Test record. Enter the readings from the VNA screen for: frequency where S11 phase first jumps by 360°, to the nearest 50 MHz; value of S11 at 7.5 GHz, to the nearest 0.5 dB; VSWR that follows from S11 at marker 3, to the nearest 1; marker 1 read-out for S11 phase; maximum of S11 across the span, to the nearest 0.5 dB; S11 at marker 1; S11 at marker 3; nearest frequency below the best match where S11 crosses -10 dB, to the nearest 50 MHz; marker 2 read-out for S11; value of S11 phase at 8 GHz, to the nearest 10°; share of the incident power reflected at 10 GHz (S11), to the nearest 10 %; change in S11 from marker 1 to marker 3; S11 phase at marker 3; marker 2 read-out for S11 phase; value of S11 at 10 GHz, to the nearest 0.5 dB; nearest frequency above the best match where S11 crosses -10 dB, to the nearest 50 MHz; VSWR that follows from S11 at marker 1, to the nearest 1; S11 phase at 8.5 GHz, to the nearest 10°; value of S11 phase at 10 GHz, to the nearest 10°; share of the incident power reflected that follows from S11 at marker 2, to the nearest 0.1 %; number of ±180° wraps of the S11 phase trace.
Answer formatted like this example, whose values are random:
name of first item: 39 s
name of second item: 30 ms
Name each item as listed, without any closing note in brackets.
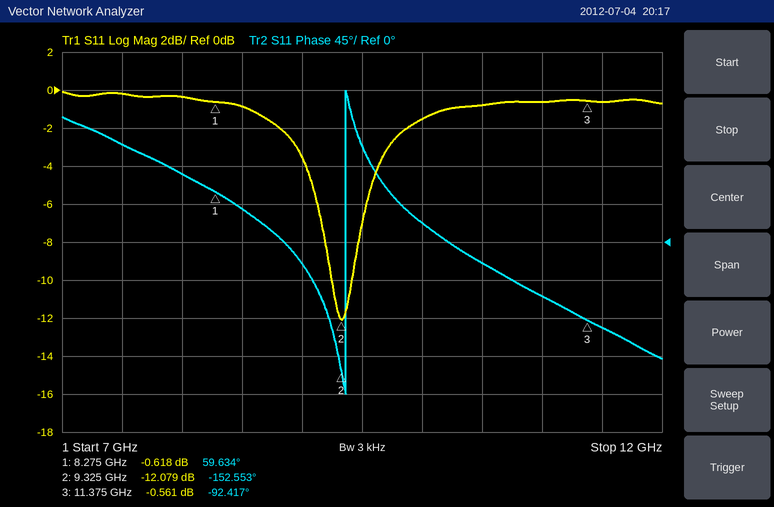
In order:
frequency where S11 phase first jumps by 360°, to the nearest 50 MHz: 9.35 GHz
value of S11 at 7.5 GHz, to the nearest 0.5 dB: 0.0 dB
VSWR that follows from S11 at marker 3, to the nearest 1: 31
marker 1 read-out for S11 phase: 59.634°
maximum of S11 across the span, to the nearest 0.5 dB: 0.0 dB
S11 at marker 1: -0.618 dB
S11 at marker 3: -0.561 dB
nearest frequency below the best match where S11 crosses -10 dB, to the nearest 50 MHz: 9.25 GHz
marker 2 read-out for S11: -12.079 dB
value of S11 phase at 8 GHz, to the nearest 10°: 80°
share of the incident power reflected at 10 GHz (S11), to the nearest 10 %: 70 %
change in S11 from marker 1 to marker 3: 0.057 dB
S11 phase at marker 3: -92.417°
marker 2 read-out for S11 phase: -152.553°
value of S11 at 10 GHz, to the nearest 0.5 dB: -1.5 dB
nearest frequency above the best match where S11 crosses -10 dB, to the nearest 50 MHz: 9.40 GHz
VSWR that follows from S11 at marker 1, to the nearest 1: 28
S11 phase at 8.5 GHz, to the nearest 10°: 40°
value of S11 phase at 10 GHz, to the nearest 10°: 20°
share of the incident power reflected that follows from S11 at marker 2, to the nearest 0.1 %: 6.2 %
number of ±180° wraps of the S11 phase trace: 1
